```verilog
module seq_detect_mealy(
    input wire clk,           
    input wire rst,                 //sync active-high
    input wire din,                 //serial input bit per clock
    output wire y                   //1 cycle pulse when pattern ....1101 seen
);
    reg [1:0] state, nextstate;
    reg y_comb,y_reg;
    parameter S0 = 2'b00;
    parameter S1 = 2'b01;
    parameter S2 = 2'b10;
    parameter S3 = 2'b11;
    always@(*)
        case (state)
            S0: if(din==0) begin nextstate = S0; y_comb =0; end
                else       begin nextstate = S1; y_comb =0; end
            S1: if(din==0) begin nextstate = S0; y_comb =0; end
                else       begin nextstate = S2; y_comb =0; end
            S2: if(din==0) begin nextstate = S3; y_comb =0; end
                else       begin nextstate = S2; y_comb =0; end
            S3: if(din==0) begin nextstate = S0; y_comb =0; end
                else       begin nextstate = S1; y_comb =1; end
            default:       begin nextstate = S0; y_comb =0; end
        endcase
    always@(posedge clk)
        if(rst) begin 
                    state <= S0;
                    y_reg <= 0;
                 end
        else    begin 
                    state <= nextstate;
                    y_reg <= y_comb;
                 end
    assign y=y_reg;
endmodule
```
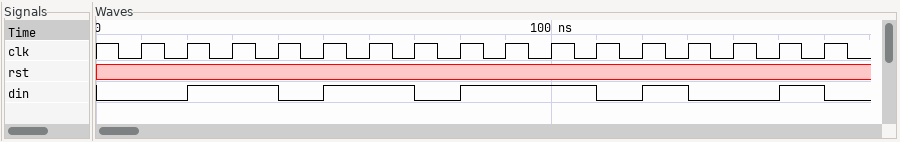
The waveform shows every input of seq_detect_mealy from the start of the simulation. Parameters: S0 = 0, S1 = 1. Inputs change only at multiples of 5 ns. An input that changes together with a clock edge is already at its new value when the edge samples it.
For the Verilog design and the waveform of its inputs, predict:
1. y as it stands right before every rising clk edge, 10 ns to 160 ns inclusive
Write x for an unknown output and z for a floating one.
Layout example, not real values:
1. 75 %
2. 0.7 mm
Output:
1. x 0 0 0 0 1 0 0 1 0 0 0 1 0 0 0
